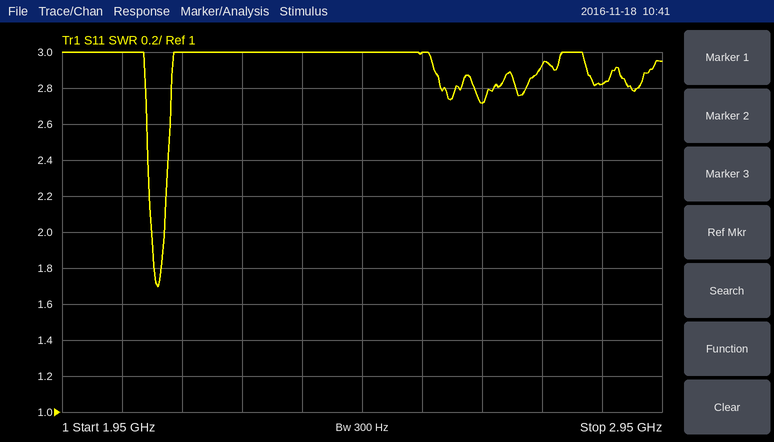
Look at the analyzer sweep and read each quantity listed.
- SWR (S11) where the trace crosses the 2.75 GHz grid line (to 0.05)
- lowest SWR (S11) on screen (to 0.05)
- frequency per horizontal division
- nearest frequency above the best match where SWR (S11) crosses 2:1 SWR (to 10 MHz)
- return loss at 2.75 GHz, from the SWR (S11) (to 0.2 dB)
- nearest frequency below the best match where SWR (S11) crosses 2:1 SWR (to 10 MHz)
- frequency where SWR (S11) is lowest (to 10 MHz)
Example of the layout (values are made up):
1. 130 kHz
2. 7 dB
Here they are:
1. 2.95
2. 1.70
3. 100 MHz
4. 2.12 GHz
5. 6.2 dB
6. 2.10 GHz
7. 2.11 GHz
